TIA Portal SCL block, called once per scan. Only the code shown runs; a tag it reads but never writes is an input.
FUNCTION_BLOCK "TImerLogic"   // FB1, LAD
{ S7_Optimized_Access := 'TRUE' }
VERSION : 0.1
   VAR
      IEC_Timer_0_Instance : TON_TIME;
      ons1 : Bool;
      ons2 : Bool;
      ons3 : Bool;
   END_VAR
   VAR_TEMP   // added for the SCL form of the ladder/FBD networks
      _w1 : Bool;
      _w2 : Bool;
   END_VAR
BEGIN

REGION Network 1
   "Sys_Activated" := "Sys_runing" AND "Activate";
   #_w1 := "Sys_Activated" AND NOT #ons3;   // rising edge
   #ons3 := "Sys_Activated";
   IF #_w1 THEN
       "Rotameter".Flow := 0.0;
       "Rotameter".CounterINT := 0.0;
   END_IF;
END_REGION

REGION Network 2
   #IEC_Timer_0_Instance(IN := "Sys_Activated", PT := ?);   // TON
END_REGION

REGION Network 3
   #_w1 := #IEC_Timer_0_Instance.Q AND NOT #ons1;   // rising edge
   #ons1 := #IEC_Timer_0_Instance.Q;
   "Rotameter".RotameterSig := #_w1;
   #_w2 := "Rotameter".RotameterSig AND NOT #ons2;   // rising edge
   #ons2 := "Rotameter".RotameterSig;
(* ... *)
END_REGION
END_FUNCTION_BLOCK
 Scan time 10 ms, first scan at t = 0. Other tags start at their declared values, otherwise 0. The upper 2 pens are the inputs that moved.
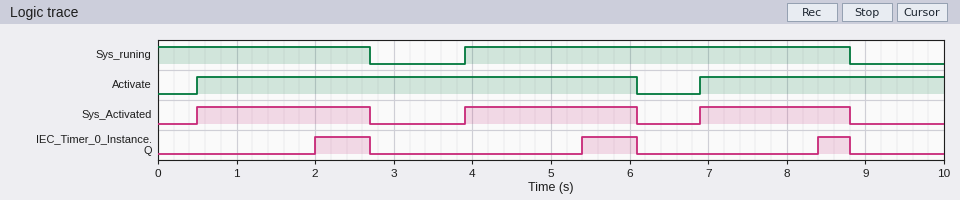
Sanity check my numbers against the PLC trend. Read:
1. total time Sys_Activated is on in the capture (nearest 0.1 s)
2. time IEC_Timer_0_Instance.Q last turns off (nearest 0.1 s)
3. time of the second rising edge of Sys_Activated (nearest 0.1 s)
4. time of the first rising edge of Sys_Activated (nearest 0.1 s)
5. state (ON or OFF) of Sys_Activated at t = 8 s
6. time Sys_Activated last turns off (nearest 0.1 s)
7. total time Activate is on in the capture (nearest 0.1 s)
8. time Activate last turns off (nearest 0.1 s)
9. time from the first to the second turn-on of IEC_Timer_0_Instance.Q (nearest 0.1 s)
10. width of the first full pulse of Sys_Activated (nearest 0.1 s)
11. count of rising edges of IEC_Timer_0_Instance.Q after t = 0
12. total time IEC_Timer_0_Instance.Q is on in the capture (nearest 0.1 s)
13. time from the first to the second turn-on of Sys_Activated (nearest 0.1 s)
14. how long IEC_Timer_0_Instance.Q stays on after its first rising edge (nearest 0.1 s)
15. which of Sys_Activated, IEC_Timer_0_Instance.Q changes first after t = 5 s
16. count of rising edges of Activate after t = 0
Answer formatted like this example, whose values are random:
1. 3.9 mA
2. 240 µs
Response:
1. 6.3 s
2. 8.8 s
3. 3.9 s
4. 0.5 s
5. ON
6. 8.8 s
7. 8.7 s
8. 6.1 s
9. 3.4 s
10. 2.2 s
11. 3
12. 1.8 s
13. 3.4 s
14. 0.7 s
15. IEC_Timer_0_Instance.Q
16. 2
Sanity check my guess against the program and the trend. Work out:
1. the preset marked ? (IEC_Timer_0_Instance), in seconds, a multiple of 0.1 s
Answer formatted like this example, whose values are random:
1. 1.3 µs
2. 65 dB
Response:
1. 1.5 s
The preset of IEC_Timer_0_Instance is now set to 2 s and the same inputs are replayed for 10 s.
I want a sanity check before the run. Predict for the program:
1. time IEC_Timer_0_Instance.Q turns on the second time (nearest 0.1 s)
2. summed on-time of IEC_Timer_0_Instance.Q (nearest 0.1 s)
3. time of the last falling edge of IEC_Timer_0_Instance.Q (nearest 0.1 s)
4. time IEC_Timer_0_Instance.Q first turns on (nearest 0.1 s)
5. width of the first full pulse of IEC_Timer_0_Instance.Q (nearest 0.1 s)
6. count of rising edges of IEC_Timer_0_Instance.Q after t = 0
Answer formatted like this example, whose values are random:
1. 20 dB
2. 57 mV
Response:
1. 5.9 s
2. 0.4 s
3. 6.1 s
4. 2.5 s
5. 0.2 s
6. 2
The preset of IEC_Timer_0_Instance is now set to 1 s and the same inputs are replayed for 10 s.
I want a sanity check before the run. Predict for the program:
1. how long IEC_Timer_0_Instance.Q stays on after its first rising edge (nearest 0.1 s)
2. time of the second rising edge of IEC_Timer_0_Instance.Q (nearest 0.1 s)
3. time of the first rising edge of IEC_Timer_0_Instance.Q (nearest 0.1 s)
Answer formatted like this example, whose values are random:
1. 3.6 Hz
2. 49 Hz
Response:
1. 1.2 s
2. 4.9 s
3. 1.5 s
